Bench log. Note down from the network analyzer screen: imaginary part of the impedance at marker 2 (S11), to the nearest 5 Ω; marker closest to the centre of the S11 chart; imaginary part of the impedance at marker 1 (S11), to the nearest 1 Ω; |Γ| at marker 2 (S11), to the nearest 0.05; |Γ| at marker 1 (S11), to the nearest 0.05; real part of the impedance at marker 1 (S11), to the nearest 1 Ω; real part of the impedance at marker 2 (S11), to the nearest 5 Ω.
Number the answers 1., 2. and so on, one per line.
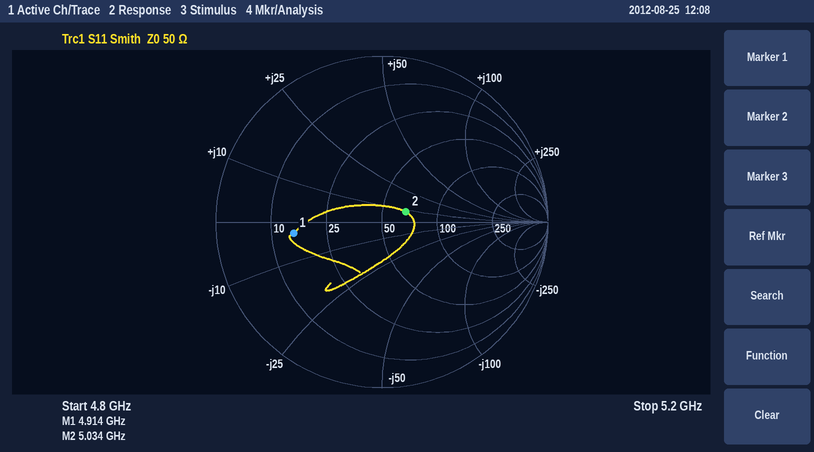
1. +10 Ω
2. marker 2
3. -3 Ω
4. 0.15
5. 0.55
6. 15 Ω
7. 65 Ω
